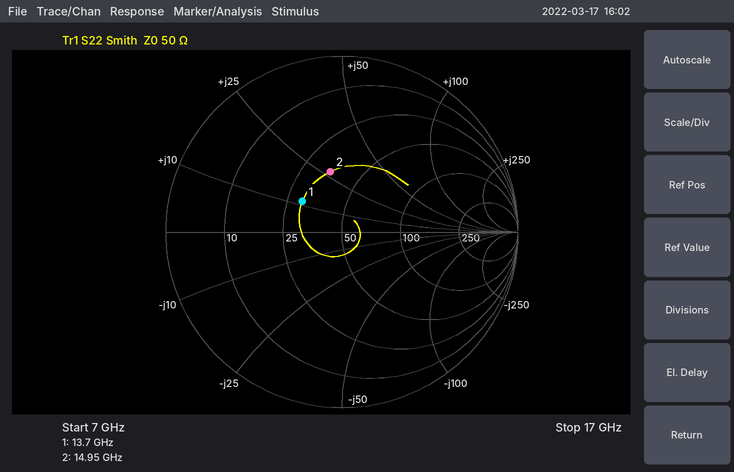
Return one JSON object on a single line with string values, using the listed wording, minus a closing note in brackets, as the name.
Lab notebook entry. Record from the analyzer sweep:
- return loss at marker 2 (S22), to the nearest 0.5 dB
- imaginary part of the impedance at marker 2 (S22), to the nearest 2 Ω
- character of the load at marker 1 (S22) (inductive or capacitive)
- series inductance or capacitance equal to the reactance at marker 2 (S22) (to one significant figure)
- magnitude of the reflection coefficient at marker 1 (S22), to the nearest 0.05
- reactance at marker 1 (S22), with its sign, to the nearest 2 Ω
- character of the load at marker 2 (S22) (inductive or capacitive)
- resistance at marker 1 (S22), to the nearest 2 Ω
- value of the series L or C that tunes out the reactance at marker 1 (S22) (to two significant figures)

{"return loss at marker 2 (S22), to the nearest 0.5 dB": "9.0 dB", "imaginary part of the impedance at marker 2 (S22), to the nearest 2 Ω": "+28 Ω", "character of the load at marker 1 (S22)": "inductive", "series inductance or capacitance equal to the reactance at marker 2 (S22)": "300 pH", "magnitude of the reflection coefficient at marker 1 (S22), to the nearest 0.05": "0.30", "reactance at marker 1 (S22), with its sign, to the nearest 2 Ω": "+12 Ω", "character of the load at marker 2 (S22)": "inductive", "resistance at marker 1 (S22), to the nearest 2 Ω": "30 Ω", "value of the series L or C that tunes out the reactance at marker 1 (S22)": "1.0 pF"}
